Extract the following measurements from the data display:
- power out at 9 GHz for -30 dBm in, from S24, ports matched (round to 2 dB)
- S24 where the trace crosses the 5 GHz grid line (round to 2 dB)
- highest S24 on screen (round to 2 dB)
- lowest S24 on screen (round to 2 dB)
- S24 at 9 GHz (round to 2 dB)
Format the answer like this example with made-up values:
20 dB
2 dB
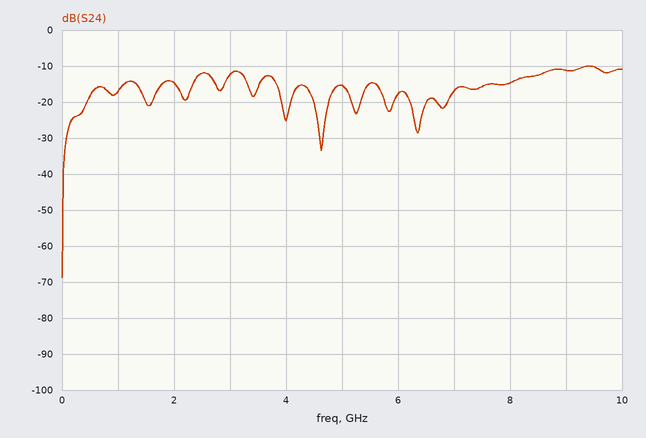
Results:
-42 dBm
-16 dB
-10 dB
-68 dB
-12 dB
